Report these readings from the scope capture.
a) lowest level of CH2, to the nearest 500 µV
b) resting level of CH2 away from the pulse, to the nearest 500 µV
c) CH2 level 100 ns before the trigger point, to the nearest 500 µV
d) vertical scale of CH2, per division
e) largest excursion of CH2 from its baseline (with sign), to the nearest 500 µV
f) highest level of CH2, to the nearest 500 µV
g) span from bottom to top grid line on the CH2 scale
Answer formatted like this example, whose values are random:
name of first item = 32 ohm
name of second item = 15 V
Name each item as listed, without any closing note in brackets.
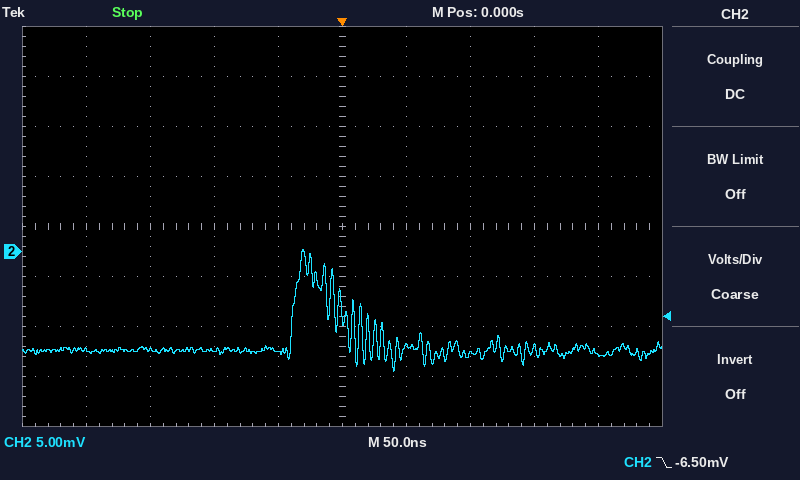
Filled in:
lowest level of CH2, to the nearest 500 µV = -12.0 mV
resting level of CH2 away from the pulse, to the nearest 500 µV = -10.0 mV
CH2 level 100 ns before the trigger point, to the nearest 500 µV = -10.0 mV
vertical scale of CH2, per division = 5 mV
largest excursion of CH2 from its baseline (with sign), to the nearest 500 µV = +10.0 mV
highest level of CH2, to the nearest 500 µV = 0.0 mV
span from bottom to top grid line on the CH2 scale = 40 mV
